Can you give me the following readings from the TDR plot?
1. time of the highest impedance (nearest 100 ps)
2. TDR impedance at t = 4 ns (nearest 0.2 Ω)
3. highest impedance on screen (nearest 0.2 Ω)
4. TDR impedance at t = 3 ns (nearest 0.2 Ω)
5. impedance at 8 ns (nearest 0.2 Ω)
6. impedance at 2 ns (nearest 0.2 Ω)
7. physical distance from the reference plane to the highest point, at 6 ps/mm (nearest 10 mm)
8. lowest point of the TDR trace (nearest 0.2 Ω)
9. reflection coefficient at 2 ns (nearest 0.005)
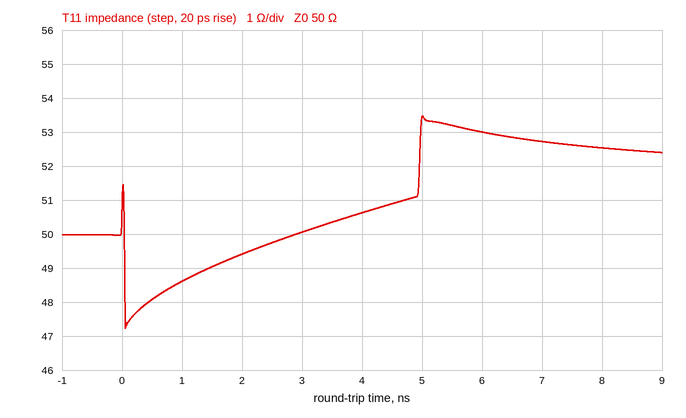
5.0 ns
50.6 Ω
53.4 Ω
50.0 Ω
52.6 Ω
49.4 Ω
420 mm
47.2 Ω
-0.005
